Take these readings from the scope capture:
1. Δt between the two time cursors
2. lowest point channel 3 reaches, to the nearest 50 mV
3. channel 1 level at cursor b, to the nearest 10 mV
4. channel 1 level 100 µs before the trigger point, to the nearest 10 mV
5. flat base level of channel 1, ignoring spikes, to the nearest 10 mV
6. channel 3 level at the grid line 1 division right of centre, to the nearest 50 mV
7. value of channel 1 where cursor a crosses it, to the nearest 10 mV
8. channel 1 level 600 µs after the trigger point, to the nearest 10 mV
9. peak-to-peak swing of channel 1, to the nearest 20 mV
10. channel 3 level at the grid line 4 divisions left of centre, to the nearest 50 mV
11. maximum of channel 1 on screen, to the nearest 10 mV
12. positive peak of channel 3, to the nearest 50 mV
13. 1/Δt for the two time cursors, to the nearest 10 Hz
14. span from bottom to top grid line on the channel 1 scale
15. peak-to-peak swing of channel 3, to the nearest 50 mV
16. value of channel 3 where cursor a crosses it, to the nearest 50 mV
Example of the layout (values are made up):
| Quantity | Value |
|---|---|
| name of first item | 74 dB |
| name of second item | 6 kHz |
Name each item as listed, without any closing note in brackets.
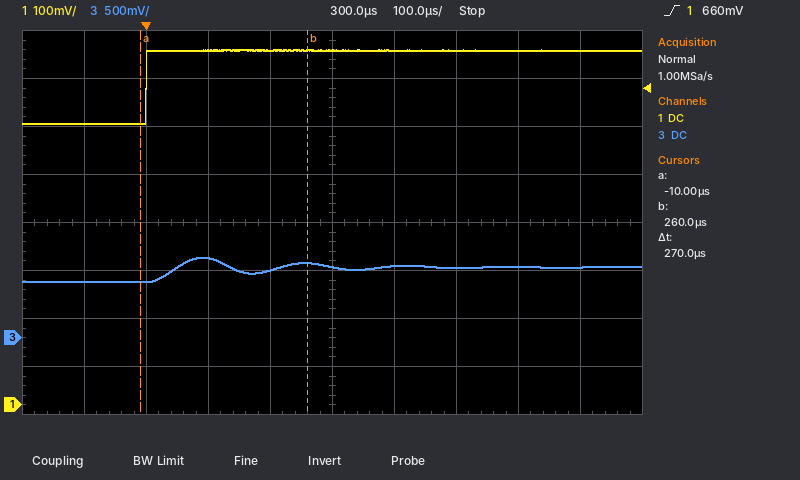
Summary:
| Quantity | Value |
|---|---|
| Δt between the two time cursors | 270 µs |
| lowest point channel 3 reaches, to the nearest 50 mV | 600 mV |
| channel 1 level at cursor b, to the nearest 10 mV | 740 mV |
| channel 1 level 100 µs before the trigger point, to the nearest 10 mV | 590 mV |
| flat base level of channel 1, ignoring spikes, to the nearest 10 mV | 590 mV |
| channel 3 level at the grid line 1 division right of centre, to the nearest 50 mV | 750 mV |
| value of channel 1 where cursor a crosses it, to the nearest 10 mV | 590 mV |
| channel 1 level 600 µs after the trigger point, to the nearest 10 mV | 740 mV |
| peak-to-peak swing of channel 1, to the nearest 20 mV | 160 mV |
| channel 3 level at the grid line 4 divisions left of centre, to the nearest 50 mV | 600 mV |
| maximum of channel 1 on screen, to the nearest 10 mV | 740 mV |
| positive peak of channel 3, to the nearest 50 mV | 850 mV |
| 1/Δt for the two time cursors, to the nearest 10 Hz | 3.70 kHz |
| span from bottom to top grid line on the channel 1 scale | 800 mV |
| peak-to-peak swing of channel 3, to the nearest 50 mV | 250 mV |
| value of channel 3 where cursor a crosses it, to the nearest 50 mV | 600 mV |
